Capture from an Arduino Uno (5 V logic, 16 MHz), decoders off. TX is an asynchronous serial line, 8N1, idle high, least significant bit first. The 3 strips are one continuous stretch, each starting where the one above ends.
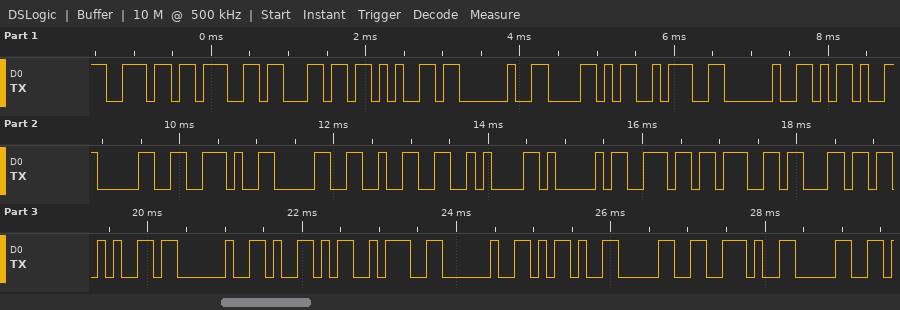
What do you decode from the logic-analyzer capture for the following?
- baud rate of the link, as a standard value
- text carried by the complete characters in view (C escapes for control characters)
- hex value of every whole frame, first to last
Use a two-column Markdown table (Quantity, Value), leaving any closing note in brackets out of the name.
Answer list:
| Quantity | Value |
|---|---|
| baud rate of the link, as a standard value | 9600 baud |
| text carried by the complete characters in view | "ngle X: -0.02\nAngle Y: -0.0" |
| hex value of every whole frame, first to last | 6E 67 6C 65 20 58 3A 20 2D 30 2E 30 32 0A 41 6E 67 6C 65 20 59 3A 20 2D 30 2E 30 |
